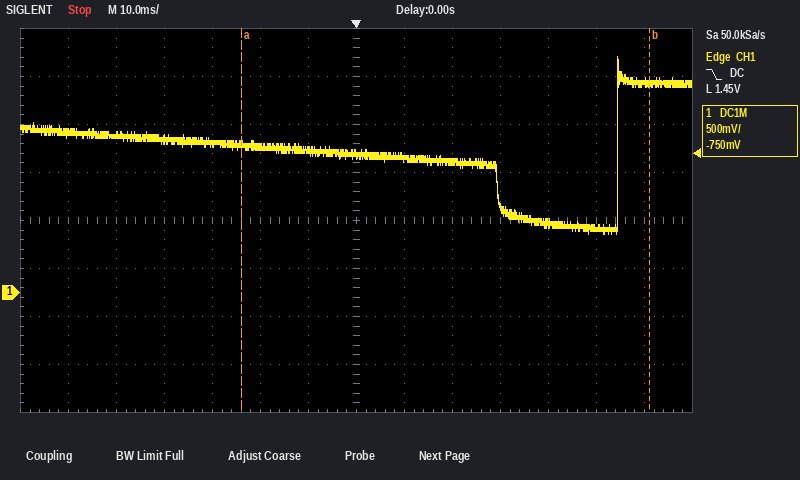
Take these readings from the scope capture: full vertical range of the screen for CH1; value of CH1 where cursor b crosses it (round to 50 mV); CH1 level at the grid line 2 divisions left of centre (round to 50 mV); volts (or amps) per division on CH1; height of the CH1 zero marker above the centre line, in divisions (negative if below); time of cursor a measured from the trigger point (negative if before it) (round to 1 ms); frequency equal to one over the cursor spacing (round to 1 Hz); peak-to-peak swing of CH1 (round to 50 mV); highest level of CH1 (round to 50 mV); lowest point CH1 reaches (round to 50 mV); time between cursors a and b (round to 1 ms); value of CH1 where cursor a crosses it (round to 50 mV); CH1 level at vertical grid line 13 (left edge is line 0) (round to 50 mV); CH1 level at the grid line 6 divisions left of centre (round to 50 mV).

4 V
2.20 V
1.50 V
500 mV
-1.5 div
-24 ms
12 Hz
1.85 V
2.45 V
600 mV
85 ms
1.55 V
2.20 V
1.65 V
